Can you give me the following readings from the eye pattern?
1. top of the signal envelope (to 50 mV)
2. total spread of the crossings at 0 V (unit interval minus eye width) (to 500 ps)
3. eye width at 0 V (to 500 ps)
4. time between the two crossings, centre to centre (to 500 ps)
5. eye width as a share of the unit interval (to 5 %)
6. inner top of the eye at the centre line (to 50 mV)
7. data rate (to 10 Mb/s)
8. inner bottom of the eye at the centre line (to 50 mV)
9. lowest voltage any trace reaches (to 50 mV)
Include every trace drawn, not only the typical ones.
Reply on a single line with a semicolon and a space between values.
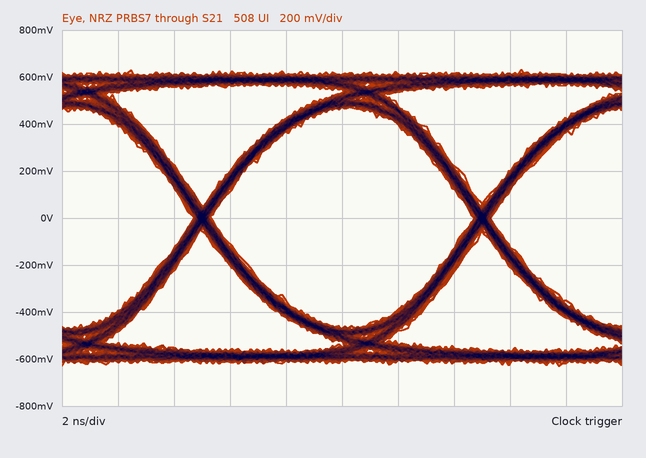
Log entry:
650 mV; 500 ps; 9.5 ns; 10.0 ns; 95 %; 450 mV; 100 Mb/s; -450 mV; -650 mV
